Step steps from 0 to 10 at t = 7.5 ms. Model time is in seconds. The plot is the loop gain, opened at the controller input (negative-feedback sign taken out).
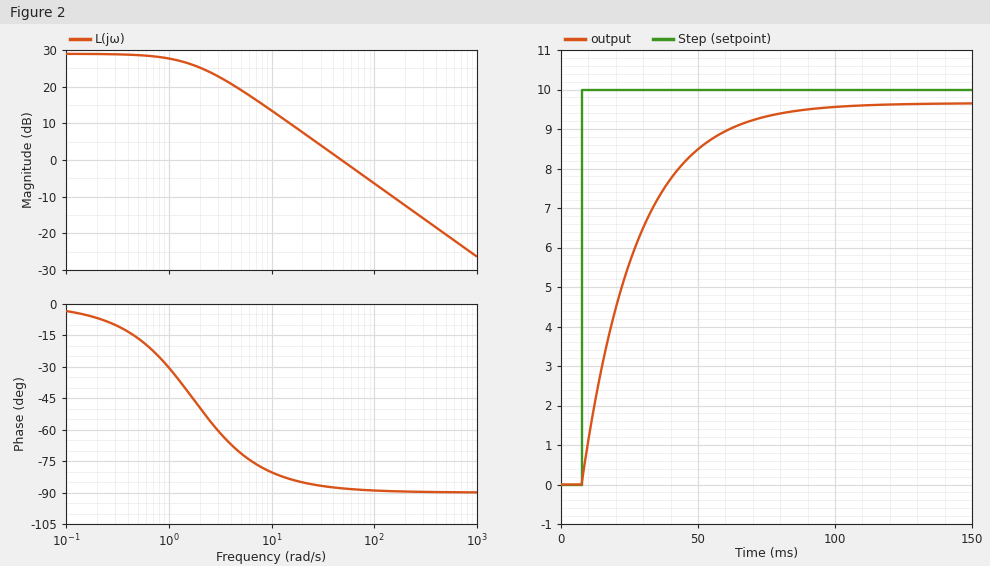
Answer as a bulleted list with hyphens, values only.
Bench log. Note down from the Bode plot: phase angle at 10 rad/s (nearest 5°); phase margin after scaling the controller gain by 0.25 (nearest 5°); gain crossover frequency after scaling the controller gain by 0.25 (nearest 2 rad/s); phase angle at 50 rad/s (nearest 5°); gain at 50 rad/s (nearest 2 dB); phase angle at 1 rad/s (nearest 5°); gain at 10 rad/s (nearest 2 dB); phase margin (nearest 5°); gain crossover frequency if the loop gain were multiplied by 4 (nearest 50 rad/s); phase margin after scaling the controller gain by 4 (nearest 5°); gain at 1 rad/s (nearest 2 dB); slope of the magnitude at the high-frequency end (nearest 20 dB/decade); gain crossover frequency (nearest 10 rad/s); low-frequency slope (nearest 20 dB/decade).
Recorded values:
- -80°
- 100°
- 12 rad/s
- -90°
- 0 dB
- -30°
- 14 dB
- 90°
- 200 rad/s
- 90°
- 28 dB
- -20 dB/decade
- 50 rad/s
- 0 dB/decade
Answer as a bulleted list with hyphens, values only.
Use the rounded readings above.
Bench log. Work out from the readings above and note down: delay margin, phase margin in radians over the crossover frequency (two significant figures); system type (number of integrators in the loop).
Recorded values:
- 0.031 s
- 0
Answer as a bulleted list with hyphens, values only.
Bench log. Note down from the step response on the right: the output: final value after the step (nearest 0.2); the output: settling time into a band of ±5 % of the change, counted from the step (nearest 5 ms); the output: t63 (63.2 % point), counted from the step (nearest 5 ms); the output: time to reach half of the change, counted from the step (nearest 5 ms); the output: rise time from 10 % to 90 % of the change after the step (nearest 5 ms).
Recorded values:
- 9.6
- 60 ms
- 20 ms
- 15 ms
- 45 ms
